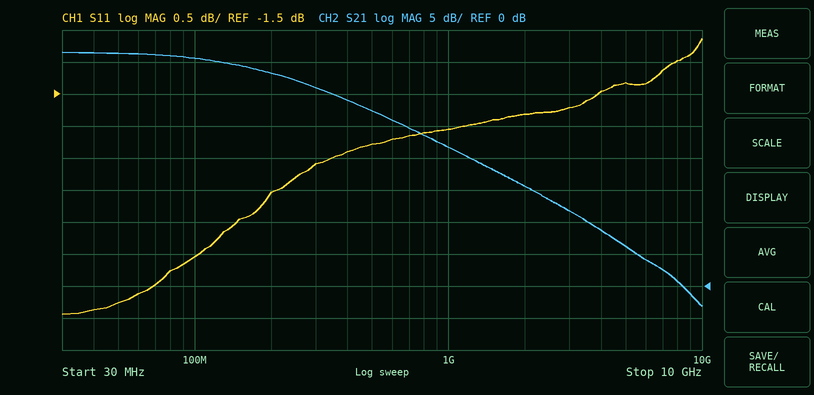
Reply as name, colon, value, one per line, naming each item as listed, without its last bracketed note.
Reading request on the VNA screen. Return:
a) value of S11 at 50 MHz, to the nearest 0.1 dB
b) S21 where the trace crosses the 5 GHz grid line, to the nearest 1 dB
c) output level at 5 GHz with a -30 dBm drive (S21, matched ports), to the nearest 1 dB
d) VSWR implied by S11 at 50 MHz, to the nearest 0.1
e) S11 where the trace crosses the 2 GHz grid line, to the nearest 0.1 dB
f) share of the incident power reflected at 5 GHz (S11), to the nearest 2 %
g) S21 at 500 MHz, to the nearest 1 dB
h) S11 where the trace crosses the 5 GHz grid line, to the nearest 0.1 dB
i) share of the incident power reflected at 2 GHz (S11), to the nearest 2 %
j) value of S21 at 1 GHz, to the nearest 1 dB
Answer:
value of S11 at 50 MHz, to the nearest 0.1 dB: -4.8 dB
S21 where the trace crosses the 5 GHz grid line, to the nearest 1 dB: 6 dB
output level at 5 GHz with a -30 dBm drive (S21, matched ports), to the nearest 1 dB: -24 dBm
VSWR implied by S11 at 50 MHz, to the nearest 0.1: 3.7
S11 where the trace crosses the 2 GHz grid line, to the nearest 0.1 dB: -1.8 dB
share of the incident power reflected at 5 GHz (S11), to the nearest 2 %: 74 %
S21 at 500 MHz, to the nearest 1 dB: 27 dB
S11 where the trace crosses the 5 GHz grid line, to the nearest 0.1 dB: -1.3 dB
share of the incident power reflected at 2 GHz (S11), to the nearest 2 %: 66 %
value of S21 at 1 GHz, to the nearest 1 dB: 22 dB
